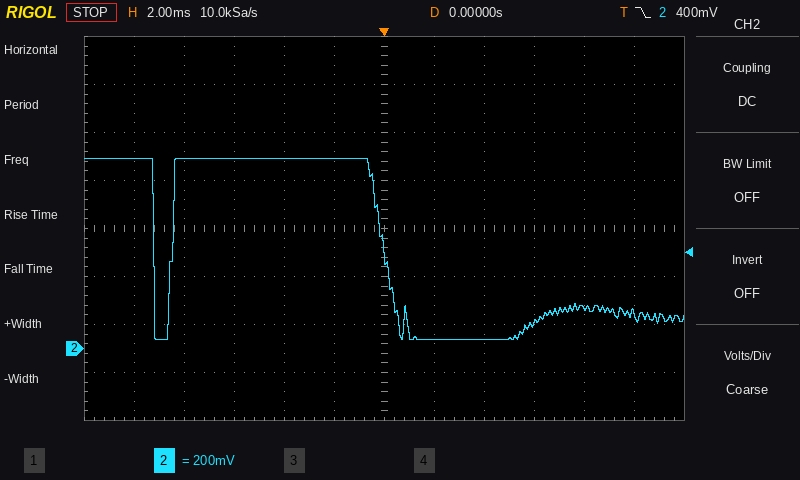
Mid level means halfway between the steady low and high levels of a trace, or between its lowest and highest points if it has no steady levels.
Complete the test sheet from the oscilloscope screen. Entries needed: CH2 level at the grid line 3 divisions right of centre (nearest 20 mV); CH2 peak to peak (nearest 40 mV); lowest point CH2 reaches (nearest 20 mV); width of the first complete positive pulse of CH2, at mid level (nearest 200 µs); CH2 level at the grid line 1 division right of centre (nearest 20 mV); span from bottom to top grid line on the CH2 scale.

100 mV
760 mV
40 mV
8.4 ms
40 mV
1.6 V
